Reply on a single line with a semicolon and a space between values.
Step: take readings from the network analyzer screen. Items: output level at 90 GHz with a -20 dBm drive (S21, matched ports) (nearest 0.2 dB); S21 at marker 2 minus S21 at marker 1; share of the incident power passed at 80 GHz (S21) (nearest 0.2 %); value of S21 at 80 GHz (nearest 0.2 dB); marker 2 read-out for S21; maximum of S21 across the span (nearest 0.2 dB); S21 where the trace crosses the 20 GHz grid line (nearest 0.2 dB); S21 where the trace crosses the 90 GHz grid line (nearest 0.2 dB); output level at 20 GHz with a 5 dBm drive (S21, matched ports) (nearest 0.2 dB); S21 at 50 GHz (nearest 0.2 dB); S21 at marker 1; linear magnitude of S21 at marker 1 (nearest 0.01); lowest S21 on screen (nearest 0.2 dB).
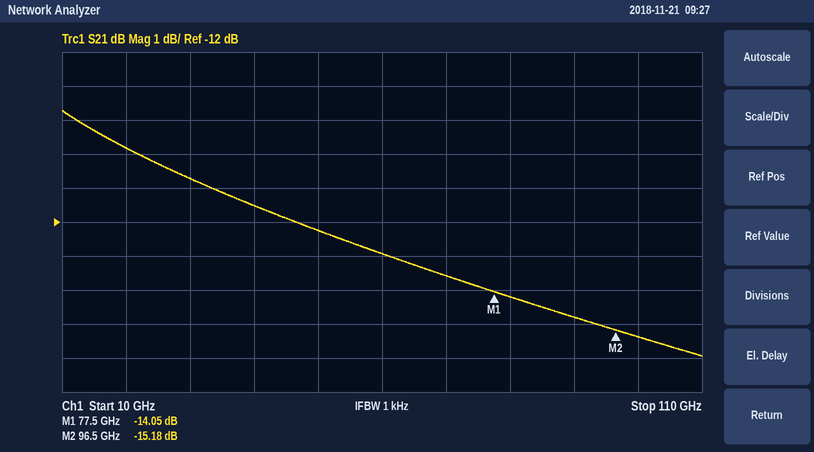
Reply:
-34.8 dBm; -1.13 dB; 3.8 %; -14.2 dB; -15.18 dB; -8.8 dB; -9.8 dB; -14.8 dB; -4.8 dBm; -12.2 dB; -14.05 dB; 0.20; -16.0 dB
